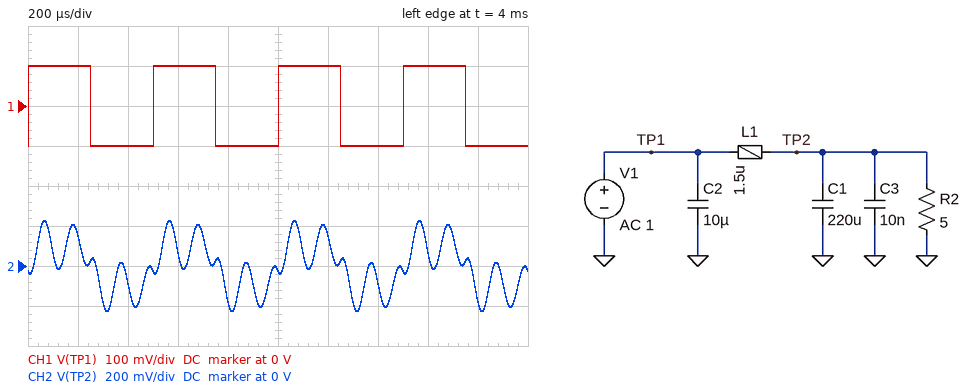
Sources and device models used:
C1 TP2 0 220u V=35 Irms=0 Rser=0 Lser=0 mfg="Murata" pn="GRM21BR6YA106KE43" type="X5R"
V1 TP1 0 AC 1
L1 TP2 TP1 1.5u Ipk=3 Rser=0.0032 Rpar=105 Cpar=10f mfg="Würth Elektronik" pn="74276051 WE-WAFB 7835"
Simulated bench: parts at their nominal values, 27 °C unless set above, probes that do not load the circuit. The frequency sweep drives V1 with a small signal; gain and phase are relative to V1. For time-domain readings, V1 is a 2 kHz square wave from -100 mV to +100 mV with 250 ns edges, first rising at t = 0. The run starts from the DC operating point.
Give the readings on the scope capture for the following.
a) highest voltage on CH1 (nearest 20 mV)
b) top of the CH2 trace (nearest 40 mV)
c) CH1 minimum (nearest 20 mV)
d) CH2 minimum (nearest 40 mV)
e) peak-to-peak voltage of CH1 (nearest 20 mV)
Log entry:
100 mV
240 mV
-100 mV
-240 mV
200 mV
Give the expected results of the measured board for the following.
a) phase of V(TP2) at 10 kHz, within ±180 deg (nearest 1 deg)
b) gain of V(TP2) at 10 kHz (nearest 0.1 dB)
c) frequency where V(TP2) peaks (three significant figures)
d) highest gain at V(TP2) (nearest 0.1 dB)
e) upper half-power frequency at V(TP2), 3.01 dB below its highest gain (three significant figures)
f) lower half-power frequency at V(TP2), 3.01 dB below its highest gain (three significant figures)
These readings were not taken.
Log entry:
-168 deg
10.2 dB
8.76 kHz
25.0 dB
9.00 kHz
8.51 kHz
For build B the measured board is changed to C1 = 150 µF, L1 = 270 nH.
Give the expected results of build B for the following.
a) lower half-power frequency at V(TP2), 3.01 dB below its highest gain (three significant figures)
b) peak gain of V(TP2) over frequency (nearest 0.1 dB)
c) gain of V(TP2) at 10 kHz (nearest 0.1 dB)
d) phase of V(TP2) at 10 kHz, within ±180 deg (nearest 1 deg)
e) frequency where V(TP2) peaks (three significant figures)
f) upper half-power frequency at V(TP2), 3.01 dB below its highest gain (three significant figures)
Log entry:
23.9 kHz
21.5 dB
1.5 dB
-2 deg
25.0 kHz
26.0 kHz
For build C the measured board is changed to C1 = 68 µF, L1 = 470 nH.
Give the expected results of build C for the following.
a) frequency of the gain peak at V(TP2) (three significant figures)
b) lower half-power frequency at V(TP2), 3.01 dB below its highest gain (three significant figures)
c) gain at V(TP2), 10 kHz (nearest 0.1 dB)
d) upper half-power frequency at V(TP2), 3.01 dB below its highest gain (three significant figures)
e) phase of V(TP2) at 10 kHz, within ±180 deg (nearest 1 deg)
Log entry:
28.1 kHz
27.3 kHz
1.2 dB
28.9 kHz
-1 deg
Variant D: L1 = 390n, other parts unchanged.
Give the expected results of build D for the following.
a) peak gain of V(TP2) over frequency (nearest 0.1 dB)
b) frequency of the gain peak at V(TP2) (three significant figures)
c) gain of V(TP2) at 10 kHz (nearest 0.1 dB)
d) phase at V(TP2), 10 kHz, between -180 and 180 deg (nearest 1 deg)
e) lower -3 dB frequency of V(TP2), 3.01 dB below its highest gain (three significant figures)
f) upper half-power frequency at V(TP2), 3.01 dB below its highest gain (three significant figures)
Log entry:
21.4 dB
17.2 kHz
3.6 dB
-4 deg
16.4 kHz
17.9 kHz
